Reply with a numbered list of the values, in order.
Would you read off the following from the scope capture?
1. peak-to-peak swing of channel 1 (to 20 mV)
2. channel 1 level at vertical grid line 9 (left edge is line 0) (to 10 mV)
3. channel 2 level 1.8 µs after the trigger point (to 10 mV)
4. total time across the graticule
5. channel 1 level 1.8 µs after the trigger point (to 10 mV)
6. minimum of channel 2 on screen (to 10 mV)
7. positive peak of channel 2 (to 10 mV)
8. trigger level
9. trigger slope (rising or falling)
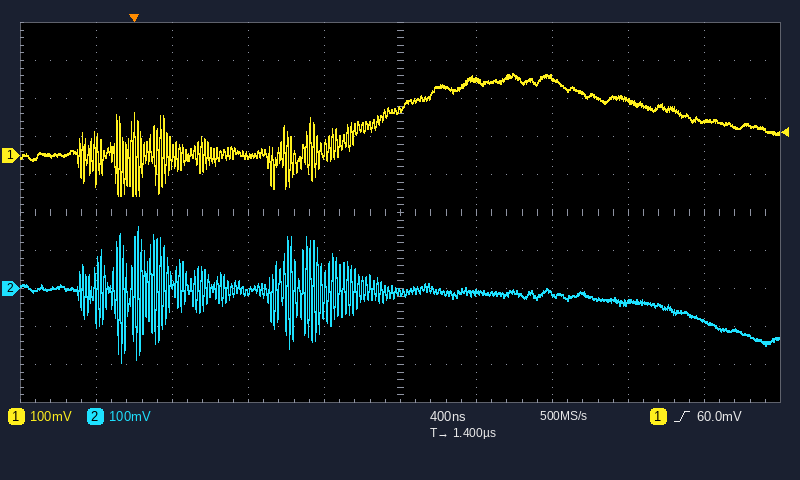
1. 320 mV
2. 90 mV
3. -10 mV
4. 4 µs
5. 200 mV
6. -190 mV
7. 160 mV
8. 60.0 mV
9. rising
